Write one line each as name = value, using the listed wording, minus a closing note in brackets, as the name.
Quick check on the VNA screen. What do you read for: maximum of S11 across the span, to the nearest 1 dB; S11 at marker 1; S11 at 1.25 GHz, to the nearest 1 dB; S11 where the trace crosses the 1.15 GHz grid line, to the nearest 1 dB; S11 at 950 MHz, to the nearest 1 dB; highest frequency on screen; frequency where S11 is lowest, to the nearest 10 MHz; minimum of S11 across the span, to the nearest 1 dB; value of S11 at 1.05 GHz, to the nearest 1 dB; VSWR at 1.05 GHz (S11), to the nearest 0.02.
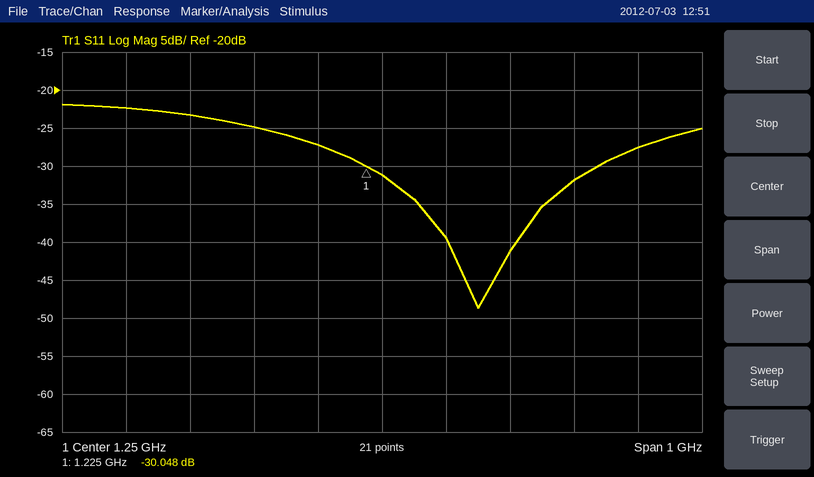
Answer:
maximum of S11 across the span, to the nearest 1 dB = -22 dB
S11 at marker 1 = -30.048 dB
S11 at 1.25 GHz, to the nearest 1 dB = -31 dB
S11 where the trace crosses the 1.15 GHz grid line, to the nearest 1 dB = -27 dB
S11 at 950 MHz, to the nearest 1 dB = -23 dB
highest frequency on screen = 1.75 GHz
frequency where S11 is lowest, to the nearest 10 MHz = 1.40 GHz
minimum of S11 across the span, to the nearest 1 dB = -49 dB
value of S11 at 1.05 GHz, to the nearest 1 dB = -25 dB
VSWR at 1.05 GHz (S11), to the nearest 0.02 = 1.12
